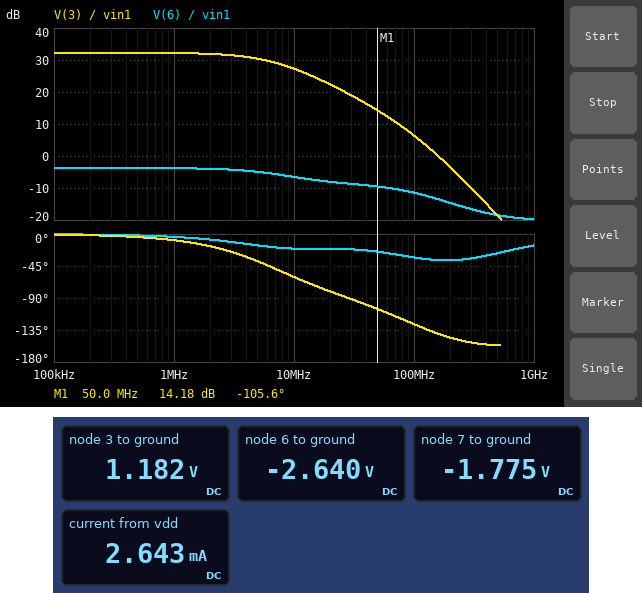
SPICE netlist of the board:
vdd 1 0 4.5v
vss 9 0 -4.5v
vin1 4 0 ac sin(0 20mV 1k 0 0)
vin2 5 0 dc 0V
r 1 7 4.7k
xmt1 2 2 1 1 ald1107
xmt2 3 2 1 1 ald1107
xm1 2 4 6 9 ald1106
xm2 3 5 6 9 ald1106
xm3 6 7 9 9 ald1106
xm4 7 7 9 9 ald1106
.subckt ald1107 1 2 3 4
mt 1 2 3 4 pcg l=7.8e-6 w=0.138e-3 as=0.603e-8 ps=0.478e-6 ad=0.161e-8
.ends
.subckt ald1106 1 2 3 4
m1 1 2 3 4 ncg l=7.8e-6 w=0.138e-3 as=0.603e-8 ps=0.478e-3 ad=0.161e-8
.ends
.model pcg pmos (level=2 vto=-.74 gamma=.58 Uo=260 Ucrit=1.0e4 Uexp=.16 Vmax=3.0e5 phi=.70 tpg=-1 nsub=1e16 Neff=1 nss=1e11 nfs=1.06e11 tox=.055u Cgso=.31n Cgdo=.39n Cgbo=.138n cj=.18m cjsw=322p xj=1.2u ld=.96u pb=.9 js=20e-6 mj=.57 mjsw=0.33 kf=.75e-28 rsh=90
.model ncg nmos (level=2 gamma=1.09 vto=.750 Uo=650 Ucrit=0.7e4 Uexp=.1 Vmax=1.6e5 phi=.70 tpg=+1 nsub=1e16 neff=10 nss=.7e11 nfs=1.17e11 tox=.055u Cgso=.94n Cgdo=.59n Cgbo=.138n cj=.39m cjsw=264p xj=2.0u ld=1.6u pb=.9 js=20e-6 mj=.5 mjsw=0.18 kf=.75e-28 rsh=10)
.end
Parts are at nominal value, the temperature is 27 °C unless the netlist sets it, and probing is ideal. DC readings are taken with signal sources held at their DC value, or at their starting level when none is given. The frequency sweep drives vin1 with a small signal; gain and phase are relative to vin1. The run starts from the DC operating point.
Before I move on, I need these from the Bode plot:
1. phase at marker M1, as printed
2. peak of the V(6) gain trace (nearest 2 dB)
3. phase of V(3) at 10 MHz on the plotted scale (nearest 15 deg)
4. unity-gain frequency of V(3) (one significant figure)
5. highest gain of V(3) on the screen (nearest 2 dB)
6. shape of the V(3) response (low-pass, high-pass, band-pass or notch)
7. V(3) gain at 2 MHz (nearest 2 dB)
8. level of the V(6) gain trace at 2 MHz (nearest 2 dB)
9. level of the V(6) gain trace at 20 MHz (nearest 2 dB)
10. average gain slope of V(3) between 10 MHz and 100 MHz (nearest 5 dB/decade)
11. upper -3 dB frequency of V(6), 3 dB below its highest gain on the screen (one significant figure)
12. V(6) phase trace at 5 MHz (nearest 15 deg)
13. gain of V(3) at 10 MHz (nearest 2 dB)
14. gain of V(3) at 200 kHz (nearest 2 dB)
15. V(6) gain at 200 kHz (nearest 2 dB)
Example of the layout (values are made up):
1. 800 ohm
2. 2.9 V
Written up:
1. -105.6 deg
2. -4 dB
3. -60 deg
4. 200 MHz
5. 32 dB
6. low-pass
7. 32 dB
8. -4 dB
9. -8 dB
10. -20 dB/decade
11. 10 MHz
12. -15 deg
13. 28 dB
14. 32 dB
15. -4 dB
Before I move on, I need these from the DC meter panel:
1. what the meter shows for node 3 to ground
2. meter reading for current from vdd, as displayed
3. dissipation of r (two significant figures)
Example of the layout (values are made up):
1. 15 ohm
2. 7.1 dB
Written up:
1. 1.182 V
2. 2.643 mA
3. 8.4 mW
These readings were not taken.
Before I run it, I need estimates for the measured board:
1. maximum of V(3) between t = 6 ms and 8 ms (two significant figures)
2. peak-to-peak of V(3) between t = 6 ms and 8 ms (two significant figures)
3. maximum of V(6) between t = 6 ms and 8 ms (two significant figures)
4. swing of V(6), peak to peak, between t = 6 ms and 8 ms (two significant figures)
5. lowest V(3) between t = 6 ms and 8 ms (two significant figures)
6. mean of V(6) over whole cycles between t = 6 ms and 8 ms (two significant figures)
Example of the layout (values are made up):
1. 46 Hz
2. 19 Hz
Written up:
1. 2.0 V
2. 1.7 V
3. -2.6 V
4. 26 mV
5. 370 mV
6. -2.6 V
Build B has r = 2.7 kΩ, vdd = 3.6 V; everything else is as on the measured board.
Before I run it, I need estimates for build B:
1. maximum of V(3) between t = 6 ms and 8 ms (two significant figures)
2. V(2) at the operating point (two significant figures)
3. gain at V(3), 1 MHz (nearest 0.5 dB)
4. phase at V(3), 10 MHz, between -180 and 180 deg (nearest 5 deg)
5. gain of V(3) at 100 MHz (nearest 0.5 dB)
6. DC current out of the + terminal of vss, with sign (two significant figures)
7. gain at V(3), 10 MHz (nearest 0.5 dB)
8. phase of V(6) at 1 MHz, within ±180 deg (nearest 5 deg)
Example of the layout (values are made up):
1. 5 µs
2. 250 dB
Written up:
1. 500 mV
2. -200 mV
3. 30.5 dB
4. -50 deg
5. 7.5 dB
6. -3.6 mA
7. 27.0 dB
8. -5 deg
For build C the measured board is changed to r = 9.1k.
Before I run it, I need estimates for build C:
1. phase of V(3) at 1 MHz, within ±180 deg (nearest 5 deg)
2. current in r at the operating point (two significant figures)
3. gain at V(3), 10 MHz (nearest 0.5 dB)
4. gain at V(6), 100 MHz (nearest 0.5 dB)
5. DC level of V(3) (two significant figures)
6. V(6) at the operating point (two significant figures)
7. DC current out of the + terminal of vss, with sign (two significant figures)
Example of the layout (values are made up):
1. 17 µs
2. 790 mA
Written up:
1. -15 deg
2. 750 µA
3. 26.0 dB
4. -12.5 dB
5. 1.9 V
6. -2.4 V
7. -1.5 mA
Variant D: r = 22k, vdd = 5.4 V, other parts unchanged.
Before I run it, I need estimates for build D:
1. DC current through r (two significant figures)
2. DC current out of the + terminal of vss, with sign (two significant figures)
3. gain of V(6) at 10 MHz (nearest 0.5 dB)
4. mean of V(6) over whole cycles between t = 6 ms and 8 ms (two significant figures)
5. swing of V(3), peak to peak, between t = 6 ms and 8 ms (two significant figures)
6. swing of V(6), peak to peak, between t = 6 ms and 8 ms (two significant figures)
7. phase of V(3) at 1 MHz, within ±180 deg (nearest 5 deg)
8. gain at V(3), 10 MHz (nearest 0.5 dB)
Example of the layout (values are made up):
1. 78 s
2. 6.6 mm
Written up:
1. 370 µA
2. -750 µA
3. -8.0 dB
4. -2.1 V
5. 2.2 V
6. 26 mV
7. -20 deg
8. 23.5 dB
